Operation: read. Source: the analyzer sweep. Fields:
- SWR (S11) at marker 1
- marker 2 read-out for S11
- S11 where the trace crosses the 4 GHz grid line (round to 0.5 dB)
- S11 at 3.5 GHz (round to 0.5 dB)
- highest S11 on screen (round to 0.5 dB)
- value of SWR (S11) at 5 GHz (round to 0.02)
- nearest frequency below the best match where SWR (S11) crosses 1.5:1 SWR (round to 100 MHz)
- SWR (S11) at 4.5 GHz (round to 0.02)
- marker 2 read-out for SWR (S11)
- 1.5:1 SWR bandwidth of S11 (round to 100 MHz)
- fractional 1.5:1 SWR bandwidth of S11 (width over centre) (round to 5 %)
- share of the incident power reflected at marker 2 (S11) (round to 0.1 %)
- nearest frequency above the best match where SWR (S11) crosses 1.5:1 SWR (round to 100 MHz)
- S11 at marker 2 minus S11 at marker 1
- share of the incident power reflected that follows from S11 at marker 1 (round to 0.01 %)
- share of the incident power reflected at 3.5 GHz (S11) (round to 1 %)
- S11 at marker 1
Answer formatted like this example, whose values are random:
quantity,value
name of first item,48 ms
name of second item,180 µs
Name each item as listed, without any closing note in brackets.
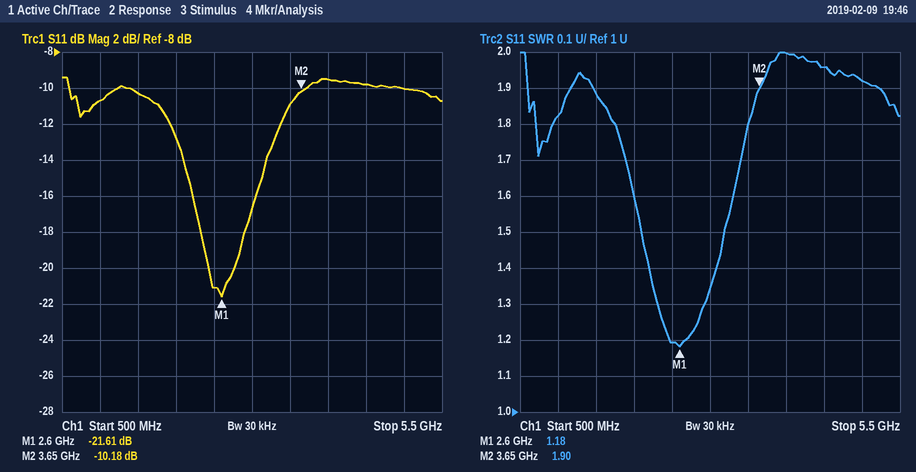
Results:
quantity,value
SWR (S11) at marker 1,1.18
marker 2 read-out for S11,-10.18 dB
S11 where the trace crosses the 4 GHz grid line,-9.5 dB
S11 at 3.5 GHz,-11.0 dB
highest S11 on screen,-9.5 dB
value of SWR (S11) at 5 GHz,1.92
nearest frequency below the best match where SWR (S11) crosses 1.5:1 SWR,2.1 GHz
SWR (S11) at 4.5 GHz,1.96
marker 2 read-out for SWR,1.90
1.5:1 SWR bandwidth of S11,1.1 GHz
fractional 1.5:1 SWR bandwidth of S11 (width over centre),40 %
share of the incident power reflected at marker 2 (S11),9.6 %
nearest frequency above the best match where SWR (S11) crosses 1.5:1 SWR,3.2 GHz
S11 at marker 2 minus S11 at marker 1,11.43 dB
share of the incident power reflected that follows from S11 at marker 1,0.69 %
share of the incident power reflected at 3.5 GHz (S11),8 %
S11 at marker 1,-21.61 dB
